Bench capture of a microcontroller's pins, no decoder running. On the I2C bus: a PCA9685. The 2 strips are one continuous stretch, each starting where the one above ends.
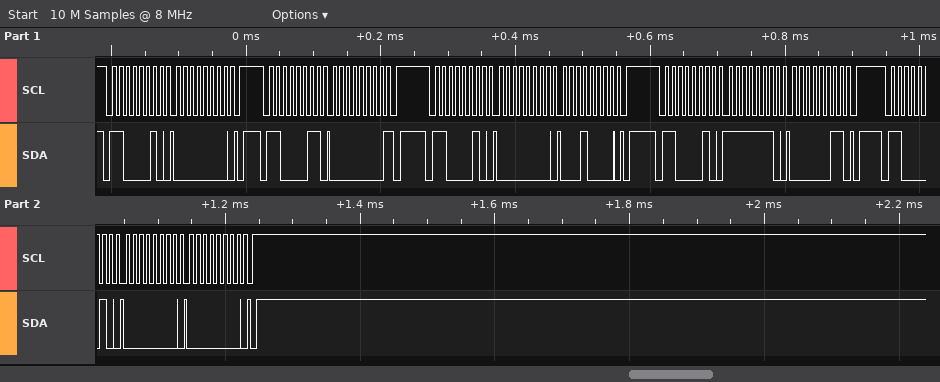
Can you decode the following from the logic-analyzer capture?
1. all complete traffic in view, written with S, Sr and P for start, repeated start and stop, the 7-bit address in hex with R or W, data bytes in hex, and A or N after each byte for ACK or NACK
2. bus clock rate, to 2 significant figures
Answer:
S 61W A 00 A P S 61R A 00 N P S 61W A 00 A 10 A P S 61W A FE A 03 A P S 61W A 00 A 00 A P
100 kHz
